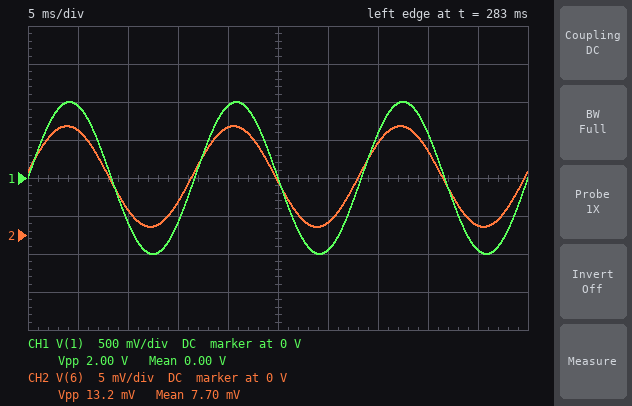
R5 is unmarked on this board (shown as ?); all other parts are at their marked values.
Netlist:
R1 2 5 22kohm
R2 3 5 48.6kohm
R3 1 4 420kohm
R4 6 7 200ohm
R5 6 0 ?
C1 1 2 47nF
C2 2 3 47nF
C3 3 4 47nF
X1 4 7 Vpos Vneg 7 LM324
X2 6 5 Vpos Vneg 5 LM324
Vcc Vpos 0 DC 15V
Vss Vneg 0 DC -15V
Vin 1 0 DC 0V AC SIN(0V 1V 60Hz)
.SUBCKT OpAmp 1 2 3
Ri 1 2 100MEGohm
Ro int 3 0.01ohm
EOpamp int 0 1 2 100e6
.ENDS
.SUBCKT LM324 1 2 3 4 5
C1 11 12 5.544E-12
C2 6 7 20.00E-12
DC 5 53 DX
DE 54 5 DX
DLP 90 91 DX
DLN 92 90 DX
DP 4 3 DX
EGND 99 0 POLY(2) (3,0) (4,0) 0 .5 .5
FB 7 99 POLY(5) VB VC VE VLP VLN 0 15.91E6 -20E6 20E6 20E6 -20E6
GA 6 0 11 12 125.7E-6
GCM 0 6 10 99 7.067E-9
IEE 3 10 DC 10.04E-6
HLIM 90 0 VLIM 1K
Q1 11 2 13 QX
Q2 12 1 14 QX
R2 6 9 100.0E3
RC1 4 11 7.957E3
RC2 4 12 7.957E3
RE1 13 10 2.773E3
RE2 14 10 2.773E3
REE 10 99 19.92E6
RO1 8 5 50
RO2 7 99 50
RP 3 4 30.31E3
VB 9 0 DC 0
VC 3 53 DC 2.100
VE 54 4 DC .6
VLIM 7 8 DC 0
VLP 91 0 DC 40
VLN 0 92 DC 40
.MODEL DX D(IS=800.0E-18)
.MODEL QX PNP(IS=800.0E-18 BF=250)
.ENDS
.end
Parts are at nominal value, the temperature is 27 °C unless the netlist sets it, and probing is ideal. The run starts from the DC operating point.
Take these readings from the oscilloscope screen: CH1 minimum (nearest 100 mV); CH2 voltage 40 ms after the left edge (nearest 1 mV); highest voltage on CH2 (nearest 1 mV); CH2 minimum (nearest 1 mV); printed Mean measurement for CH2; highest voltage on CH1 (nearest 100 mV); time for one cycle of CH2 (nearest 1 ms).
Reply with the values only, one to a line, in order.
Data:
-1.0 V
11 mV
14 mV
1 mV
7.70 mV
1.0 V
17 ms
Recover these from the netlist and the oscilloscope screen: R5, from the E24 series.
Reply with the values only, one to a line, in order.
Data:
2.4 kΩ
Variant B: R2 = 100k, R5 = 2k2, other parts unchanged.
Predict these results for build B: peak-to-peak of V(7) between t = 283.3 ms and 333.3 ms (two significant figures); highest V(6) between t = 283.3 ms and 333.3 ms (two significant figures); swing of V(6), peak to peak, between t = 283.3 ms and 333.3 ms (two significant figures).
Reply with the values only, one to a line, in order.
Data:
1.0 V
470 mV
930 mV
